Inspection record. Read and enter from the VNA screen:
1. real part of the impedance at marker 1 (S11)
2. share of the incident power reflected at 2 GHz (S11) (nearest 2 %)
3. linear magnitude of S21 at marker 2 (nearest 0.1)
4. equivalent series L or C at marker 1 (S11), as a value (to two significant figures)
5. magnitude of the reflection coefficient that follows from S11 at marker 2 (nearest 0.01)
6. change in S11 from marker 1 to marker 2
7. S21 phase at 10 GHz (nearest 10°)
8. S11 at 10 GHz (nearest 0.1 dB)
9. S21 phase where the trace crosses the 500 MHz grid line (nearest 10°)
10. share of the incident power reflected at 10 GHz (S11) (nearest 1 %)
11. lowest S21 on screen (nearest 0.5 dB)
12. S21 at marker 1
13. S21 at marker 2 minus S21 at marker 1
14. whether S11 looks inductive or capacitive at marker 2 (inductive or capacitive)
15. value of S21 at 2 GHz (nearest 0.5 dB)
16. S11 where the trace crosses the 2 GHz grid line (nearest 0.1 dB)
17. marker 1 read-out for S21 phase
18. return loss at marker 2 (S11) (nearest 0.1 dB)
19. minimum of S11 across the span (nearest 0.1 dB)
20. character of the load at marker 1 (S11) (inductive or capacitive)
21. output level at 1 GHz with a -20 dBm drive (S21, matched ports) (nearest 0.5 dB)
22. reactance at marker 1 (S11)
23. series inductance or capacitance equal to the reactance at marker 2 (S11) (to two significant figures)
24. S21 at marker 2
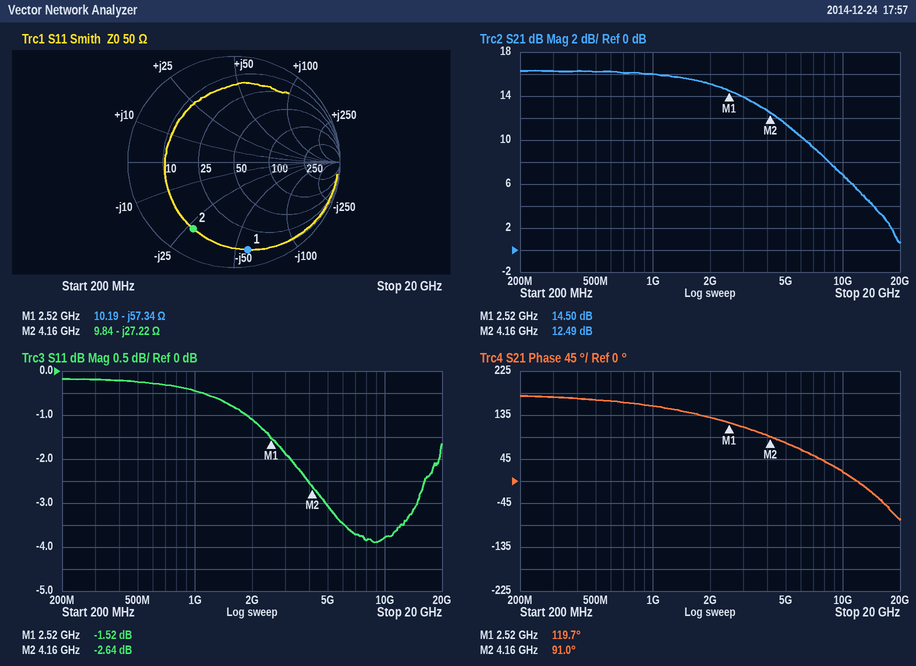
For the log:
10.19 Ω
78 %
4.2
1.1 pF
0.74
-1.12 dB
20°
-3.8 dB
170°
42 %
0.5 dB
14.50 dB
-2.01 dB
capacitive
15.0 dB
-1.1 dB
119.7°
2.6 dB
-3.9 dB
capacitive
-4.0 dBm
-57.34 Ω
1.4 pF
12.49 dB
